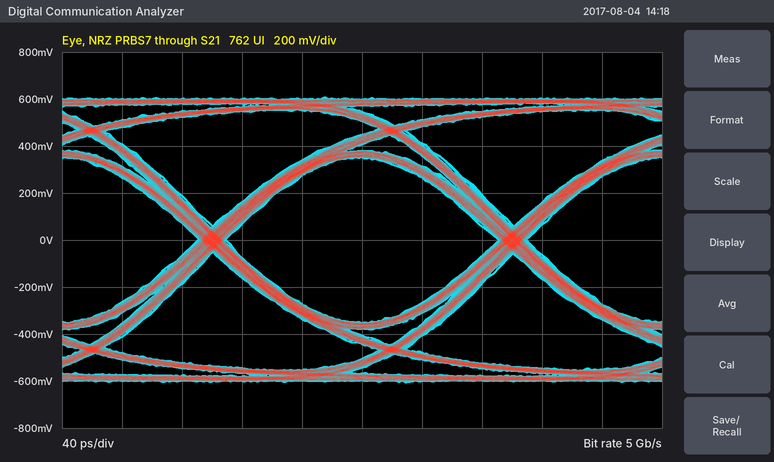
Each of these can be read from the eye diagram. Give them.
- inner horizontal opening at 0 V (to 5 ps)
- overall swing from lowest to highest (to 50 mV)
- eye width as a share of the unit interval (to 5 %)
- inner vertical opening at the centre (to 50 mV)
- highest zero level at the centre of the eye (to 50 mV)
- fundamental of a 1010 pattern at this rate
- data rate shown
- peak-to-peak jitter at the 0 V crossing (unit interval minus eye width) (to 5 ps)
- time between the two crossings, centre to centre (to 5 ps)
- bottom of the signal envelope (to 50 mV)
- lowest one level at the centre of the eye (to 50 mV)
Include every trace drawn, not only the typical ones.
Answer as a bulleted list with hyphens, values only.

- 180 ps
- 1.20 V
- 90 %
- 700 mV
- -350 mV
- 2.5 GHz
- 5 Gb/s
- 20 ps
- 200 ps
- -600 mV
- 350 mV
